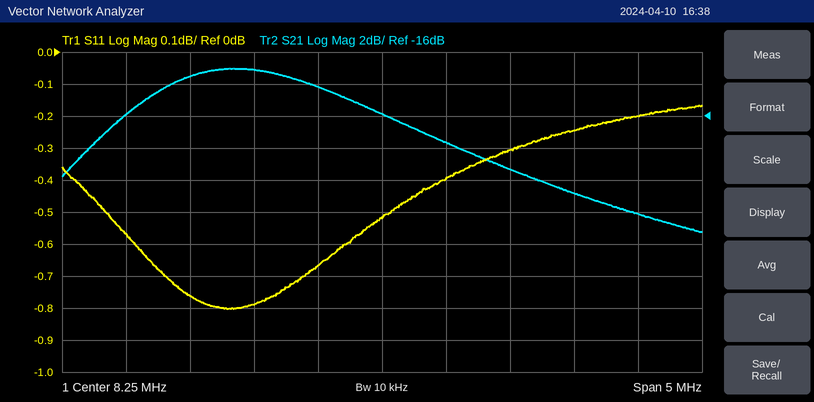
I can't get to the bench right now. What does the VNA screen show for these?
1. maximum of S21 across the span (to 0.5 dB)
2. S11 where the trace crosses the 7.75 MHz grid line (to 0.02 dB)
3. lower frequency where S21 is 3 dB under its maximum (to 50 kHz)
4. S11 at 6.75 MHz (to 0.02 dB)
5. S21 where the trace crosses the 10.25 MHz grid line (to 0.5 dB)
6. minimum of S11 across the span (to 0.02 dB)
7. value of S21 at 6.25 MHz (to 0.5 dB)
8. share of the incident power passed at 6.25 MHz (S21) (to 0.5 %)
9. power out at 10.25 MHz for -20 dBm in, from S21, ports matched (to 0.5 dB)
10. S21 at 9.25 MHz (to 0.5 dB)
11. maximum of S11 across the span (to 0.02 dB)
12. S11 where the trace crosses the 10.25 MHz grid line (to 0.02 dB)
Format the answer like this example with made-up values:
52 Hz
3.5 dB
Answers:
-13.0 dB
-0.66 dB
6.25 MHz
-0.76 dB
-22.0 dB
-0.80 dB
-16.0 dB
2.5 %
-42.0 dBm
-19.5 dB
-0.16 dB
-0.20 dB
